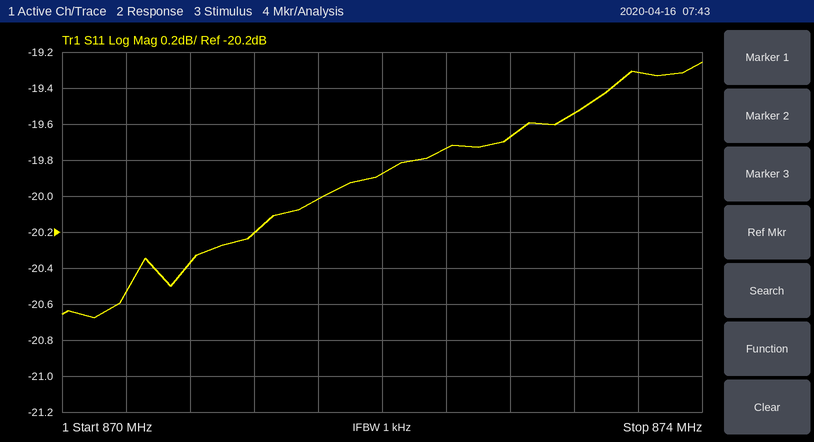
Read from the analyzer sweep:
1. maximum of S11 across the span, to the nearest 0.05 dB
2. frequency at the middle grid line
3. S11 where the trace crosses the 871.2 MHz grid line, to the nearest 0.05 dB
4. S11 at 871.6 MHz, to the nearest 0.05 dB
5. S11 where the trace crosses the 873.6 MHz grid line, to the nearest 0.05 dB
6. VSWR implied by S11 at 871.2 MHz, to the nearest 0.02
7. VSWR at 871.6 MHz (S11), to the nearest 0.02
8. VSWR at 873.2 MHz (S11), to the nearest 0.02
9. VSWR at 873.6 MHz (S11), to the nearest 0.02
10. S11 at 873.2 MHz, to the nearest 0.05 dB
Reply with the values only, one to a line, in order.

-19.25 dB
872 MHz
-20.20 dB
-20.00 dB
-19.30 dB
1.22
1.22
1.24
1.24
-19.55 dB
